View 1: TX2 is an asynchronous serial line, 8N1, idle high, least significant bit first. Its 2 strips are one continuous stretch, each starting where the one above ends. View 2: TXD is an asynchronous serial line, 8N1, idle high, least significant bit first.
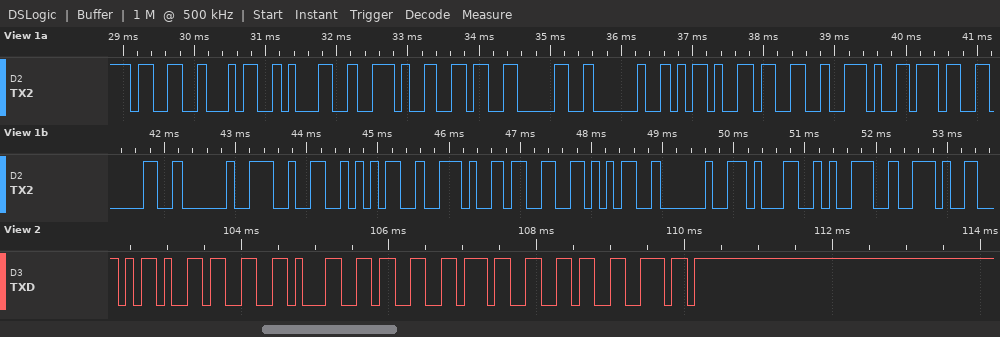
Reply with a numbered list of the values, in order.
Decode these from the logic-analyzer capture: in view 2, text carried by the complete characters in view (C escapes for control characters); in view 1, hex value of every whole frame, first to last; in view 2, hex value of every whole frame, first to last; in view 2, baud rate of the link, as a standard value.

1. "-31376n"
2. 33 34 31 2E 36 30 20 2D 33 2E 37 30 20 32 35 2E 33 35 20 31 39 2E
3. 2D 33 31 33 37 36 6E
4. 9600 baud
